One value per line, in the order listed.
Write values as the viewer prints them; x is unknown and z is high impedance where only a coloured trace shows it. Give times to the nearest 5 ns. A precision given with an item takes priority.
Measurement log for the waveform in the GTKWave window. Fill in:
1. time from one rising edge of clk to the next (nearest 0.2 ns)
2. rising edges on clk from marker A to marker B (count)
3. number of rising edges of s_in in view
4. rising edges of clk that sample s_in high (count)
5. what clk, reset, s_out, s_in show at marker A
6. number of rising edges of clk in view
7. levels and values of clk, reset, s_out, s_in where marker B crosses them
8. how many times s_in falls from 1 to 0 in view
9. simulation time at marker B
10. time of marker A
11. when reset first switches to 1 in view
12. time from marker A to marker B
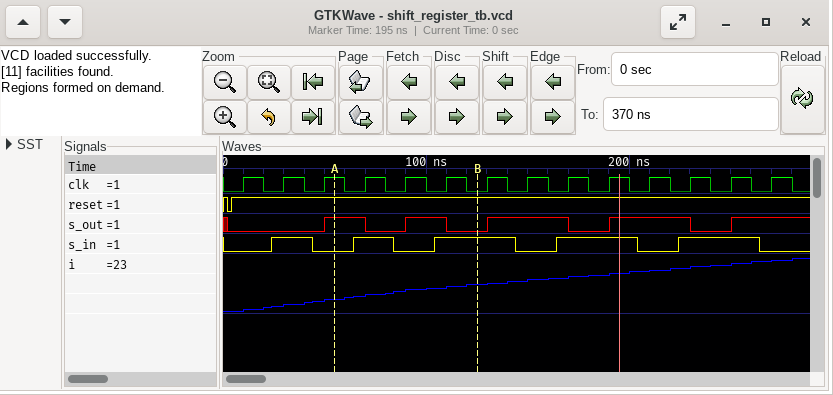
20 ns
3
5
8
clk=1, reset=1, s_out=1, s_in=0
14
clk=0, reset=1, s_out=0, s_in=1
5
125 ns
55 ns
5 ns
70 ns
